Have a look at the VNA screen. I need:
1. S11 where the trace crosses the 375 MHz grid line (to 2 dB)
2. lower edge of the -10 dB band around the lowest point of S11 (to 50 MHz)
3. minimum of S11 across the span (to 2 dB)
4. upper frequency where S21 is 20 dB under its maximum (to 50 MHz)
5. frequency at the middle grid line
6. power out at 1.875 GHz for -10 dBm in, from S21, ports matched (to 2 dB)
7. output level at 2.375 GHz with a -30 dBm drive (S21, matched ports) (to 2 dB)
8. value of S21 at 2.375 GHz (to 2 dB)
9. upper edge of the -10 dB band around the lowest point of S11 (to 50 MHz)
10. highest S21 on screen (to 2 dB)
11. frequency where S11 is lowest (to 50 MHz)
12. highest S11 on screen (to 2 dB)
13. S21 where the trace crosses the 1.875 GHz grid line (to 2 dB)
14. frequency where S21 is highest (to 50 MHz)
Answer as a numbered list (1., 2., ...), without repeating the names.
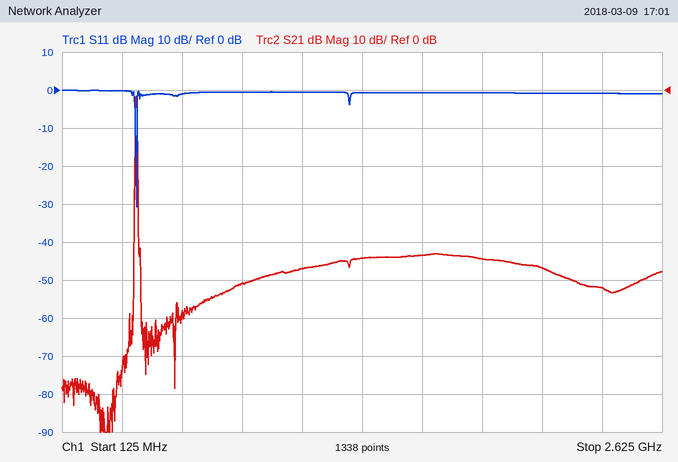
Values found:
1. 0 dB
2. 450 MHz
3. -30 dB
4. 450 MHz
5. 1.375 GHz
6. -54 dBm
7. -82 dBm
8. -52 dB
9. 450 MHz
10. -2 dB
11. 450 MHz
12. 0 dB
13. -44 dB
14. 450 MHz
